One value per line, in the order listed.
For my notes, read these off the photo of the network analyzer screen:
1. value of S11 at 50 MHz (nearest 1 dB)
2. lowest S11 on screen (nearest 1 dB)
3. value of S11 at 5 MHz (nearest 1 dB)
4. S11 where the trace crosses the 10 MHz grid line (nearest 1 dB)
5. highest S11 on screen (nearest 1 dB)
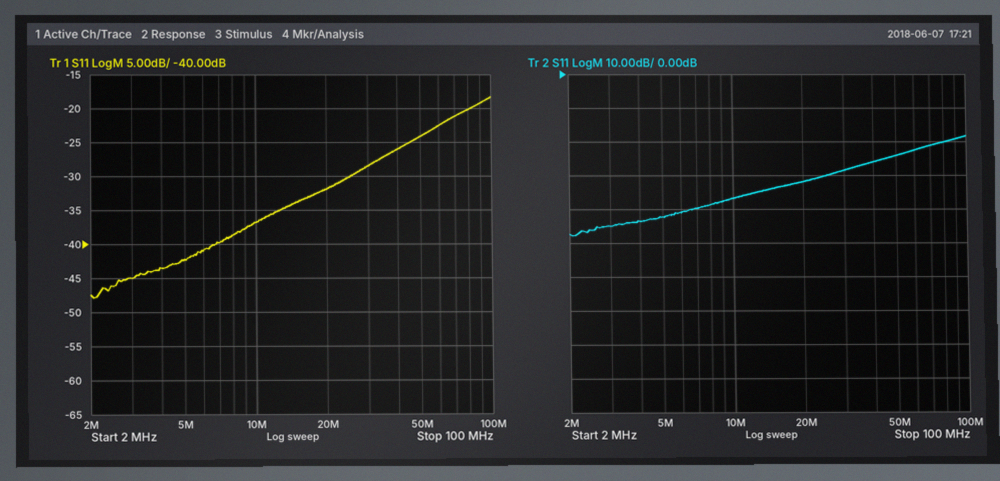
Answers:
-24 dB
-48 dB
-42 dB
-37 dB
-18 dB
